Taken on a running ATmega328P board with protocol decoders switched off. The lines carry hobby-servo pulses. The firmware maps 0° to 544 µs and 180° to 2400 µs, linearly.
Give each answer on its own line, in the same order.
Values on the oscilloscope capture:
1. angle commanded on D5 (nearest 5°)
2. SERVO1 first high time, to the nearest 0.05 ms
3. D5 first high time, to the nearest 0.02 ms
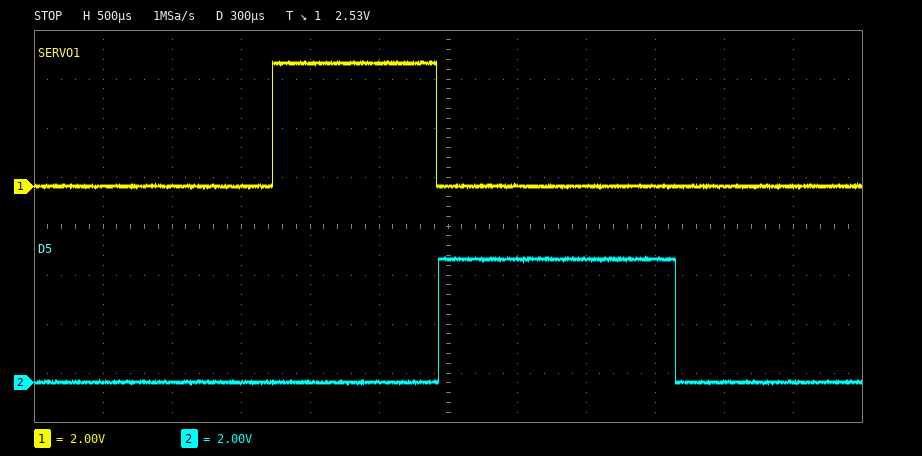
115°
1.20 ms
1.72 ms
